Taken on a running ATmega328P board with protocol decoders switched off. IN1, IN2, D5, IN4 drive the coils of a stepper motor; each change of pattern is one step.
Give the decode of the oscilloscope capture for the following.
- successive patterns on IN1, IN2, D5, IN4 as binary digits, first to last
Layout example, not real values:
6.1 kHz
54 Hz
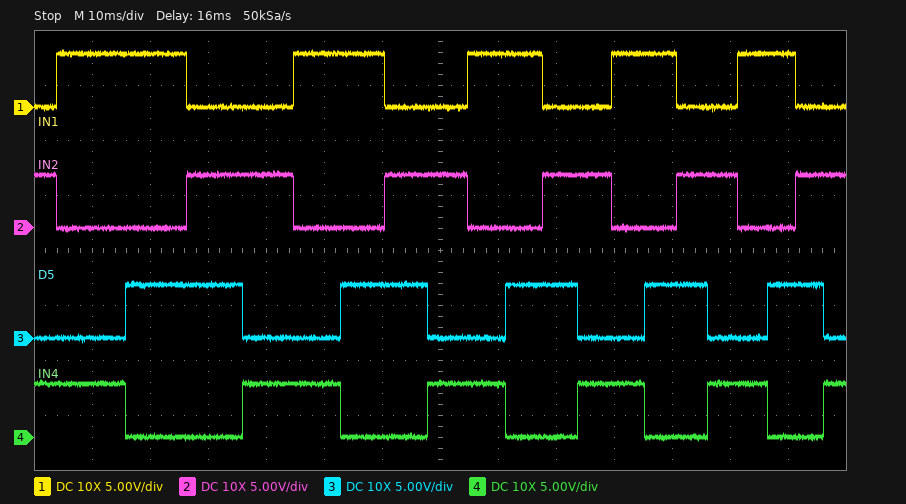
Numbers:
0101 1001 1010 0110 0101 1001 1010 0110 0101 1001 1010 0110 0101 1001 1010 0110 0101 1001 1010 0110 0101
